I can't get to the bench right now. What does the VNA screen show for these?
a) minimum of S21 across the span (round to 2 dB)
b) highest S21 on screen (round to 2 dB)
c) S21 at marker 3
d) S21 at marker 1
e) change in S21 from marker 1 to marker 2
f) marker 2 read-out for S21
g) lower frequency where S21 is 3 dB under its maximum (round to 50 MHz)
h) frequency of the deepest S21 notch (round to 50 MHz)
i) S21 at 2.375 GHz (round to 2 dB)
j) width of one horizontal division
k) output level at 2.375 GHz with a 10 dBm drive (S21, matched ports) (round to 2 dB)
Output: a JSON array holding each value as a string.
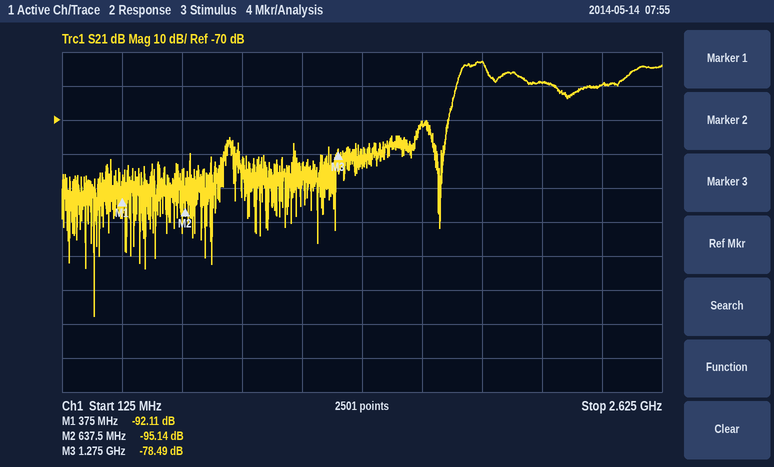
["-128 dB", "-52 dB", "-78.49 dB", "-92.11 dB", "-3.03 dB", "-95.14 dB", "1.80 GHz", "250 MHz", "-60 dB", "250 MHz", "-50 dBm"]
